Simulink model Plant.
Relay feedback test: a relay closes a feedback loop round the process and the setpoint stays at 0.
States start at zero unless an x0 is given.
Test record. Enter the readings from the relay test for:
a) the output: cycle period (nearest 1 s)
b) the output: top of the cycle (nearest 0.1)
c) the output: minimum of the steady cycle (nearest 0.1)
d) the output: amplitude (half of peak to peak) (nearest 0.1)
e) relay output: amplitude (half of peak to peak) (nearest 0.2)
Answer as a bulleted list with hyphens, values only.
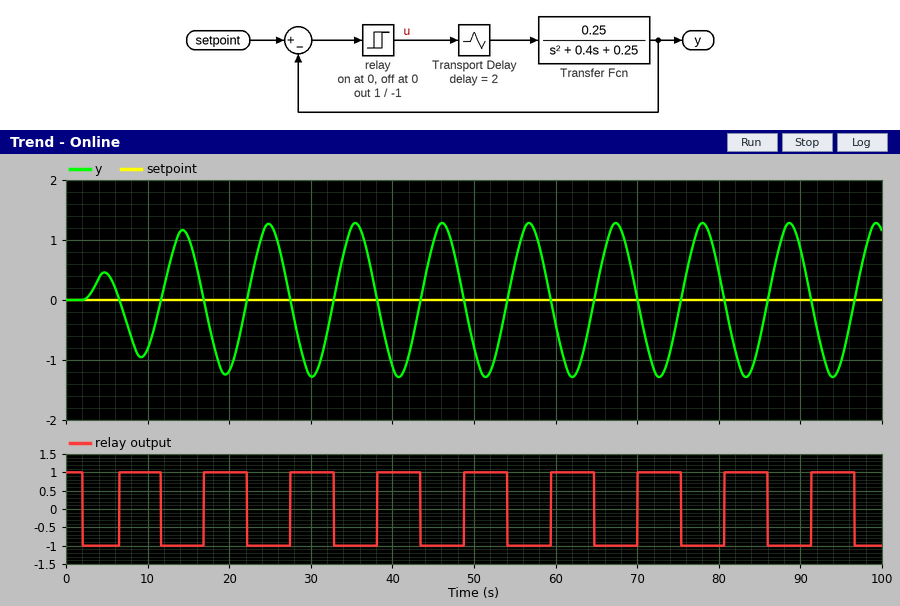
- 11 s
- 1.3
- -1.3
- 1.3
- 1.0
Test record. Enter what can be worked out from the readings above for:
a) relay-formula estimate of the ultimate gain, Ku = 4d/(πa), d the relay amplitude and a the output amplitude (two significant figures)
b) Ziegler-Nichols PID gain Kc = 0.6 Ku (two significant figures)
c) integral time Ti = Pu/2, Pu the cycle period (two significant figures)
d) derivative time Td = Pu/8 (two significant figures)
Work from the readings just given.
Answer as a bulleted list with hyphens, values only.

- 0.98
- 0.59
- 5.5 s
- 1.4 s
